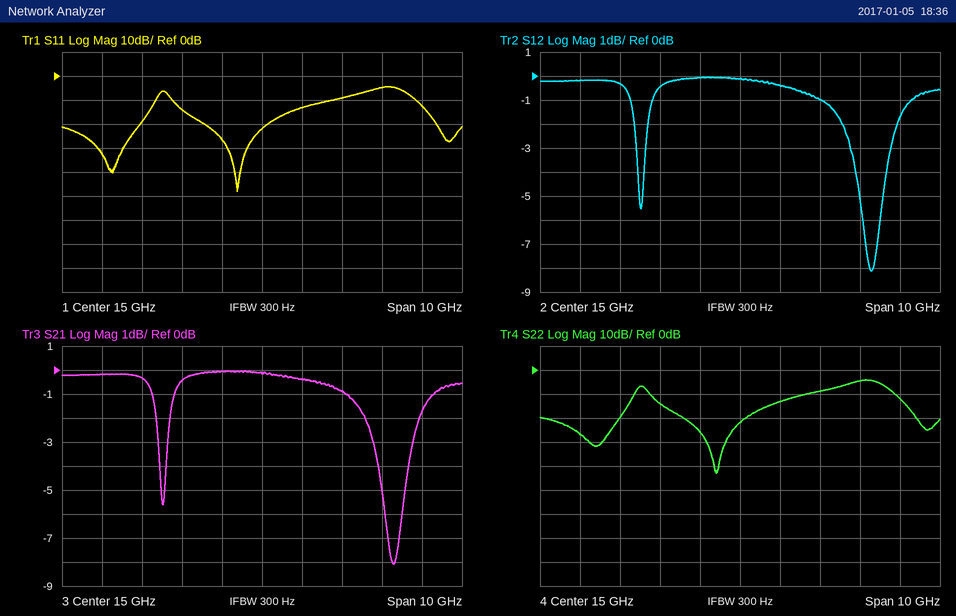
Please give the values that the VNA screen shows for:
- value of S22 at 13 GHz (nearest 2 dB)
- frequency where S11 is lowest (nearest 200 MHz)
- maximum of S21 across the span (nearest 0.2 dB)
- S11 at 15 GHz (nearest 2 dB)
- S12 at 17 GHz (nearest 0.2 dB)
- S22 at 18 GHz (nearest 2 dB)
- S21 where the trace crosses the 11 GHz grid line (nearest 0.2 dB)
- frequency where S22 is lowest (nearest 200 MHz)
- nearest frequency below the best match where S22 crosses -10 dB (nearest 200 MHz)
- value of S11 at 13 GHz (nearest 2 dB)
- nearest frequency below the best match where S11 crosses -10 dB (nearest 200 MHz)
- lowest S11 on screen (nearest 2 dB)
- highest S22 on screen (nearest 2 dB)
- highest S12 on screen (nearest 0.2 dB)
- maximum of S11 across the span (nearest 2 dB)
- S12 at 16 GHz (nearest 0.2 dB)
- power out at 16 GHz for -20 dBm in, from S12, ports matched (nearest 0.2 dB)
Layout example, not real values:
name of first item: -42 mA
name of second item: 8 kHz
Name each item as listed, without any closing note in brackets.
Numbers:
value of S22 at 13 GHz: -14 dB
frequency where S11 is lowest: 14.4 GHz
maximum of S21 across the span: 0.0 dB
S11 at 15 GHz: -22 dB
S12 at 17 GHz: -1.0 dB
S22 at 18 GHz: -4 dB
S21 where the trace crosses the 11 GHz grid line: -0.2 dB
frequency where S22 is lowest: 14.4 GHz
nearest frequency below the best match where S22 crosses -10 dB: 12.8 GHz
value of S11 at 13 GHz: -14 dB
nearest frequency below the best match where S11 crosses -10 dB: 12.8 GHz
lowest S11 on screen: -48 dB
highest S22 on screen: -4 dB
highest S12 on screen: 0.0 dB
maximum of S11 across the span: -4 dB
S12 at 16 GHz: -0.4 dB
power out at 16 GHz for -20 dBm in, from S12, ports matched: -20.4 dBm
